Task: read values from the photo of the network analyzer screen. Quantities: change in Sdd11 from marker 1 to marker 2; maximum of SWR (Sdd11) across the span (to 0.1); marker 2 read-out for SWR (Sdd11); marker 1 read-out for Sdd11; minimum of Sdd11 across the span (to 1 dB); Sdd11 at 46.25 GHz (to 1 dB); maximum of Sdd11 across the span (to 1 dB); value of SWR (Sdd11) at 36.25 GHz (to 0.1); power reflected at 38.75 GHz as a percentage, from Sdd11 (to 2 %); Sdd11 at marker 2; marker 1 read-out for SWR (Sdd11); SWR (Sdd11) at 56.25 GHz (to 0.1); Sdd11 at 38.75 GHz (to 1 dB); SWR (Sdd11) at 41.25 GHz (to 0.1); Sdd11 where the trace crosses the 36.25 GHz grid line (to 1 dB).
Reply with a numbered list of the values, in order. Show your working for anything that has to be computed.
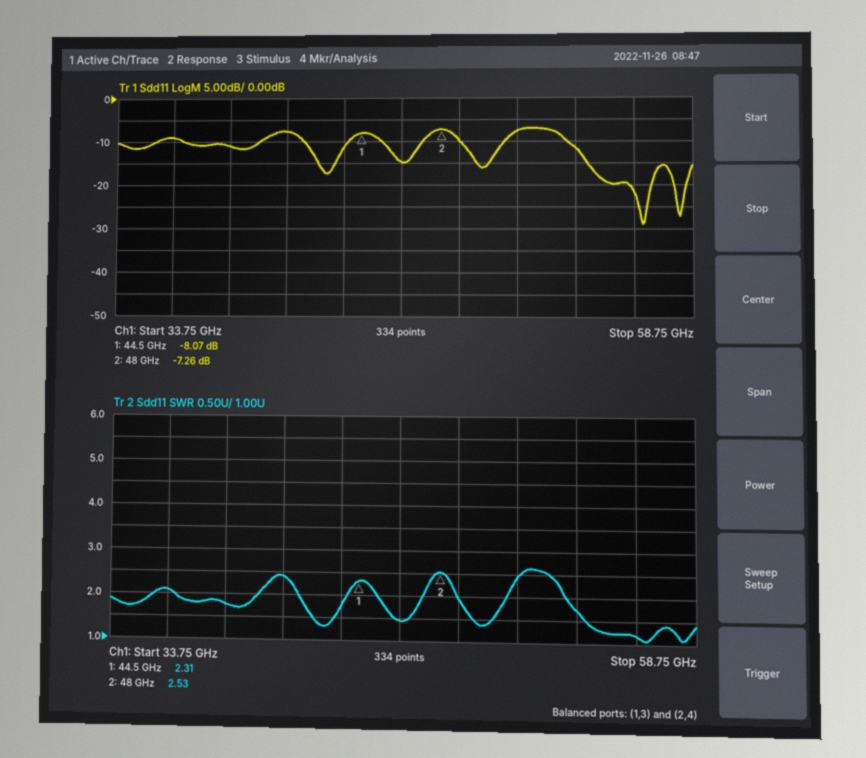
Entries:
1. -7.26 − (-8.07) = 0.81 dB
2. 2.6
3. 2.53
4. -8.07 dB
5. -29 dB
6. -15 dB
7. -7 dB
8. 2.1
9. 10^(-11/10) ≈ 8 %
10. -7.26 dB
11. 2.31
12. 1.2
13. -11 dB
14. 2.4
15. -9 dB
